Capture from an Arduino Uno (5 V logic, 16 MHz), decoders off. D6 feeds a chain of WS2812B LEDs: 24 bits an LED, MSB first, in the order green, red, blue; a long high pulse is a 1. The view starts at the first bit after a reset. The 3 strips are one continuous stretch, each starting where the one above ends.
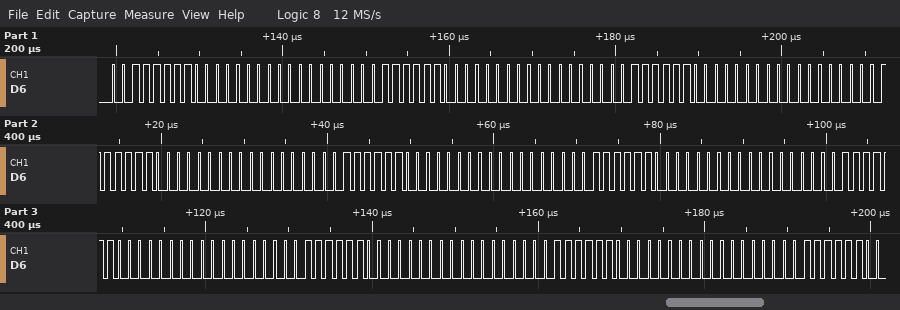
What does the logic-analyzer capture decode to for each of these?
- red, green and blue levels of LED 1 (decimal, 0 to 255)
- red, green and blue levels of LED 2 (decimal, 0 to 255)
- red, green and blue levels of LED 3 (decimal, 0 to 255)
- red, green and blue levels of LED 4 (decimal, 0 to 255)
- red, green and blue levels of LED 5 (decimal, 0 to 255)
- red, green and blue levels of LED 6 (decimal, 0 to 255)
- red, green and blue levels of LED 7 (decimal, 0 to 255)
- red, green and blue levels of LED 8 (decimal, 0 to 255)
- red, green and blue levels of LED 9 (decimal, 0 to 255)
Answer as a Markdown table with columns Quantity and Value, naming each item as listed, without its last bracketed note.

| Quantity | Value |
|---|---|
| red, green and blue levels of LED 1 | 0, 63, 0 |
| red, green and blue levels of LED 2 | 0, 63, 0 |
| red, green and blue levels of LED 3 | 0, 63, 0 |
| red, green and blue levels of LED 4 | 0, 63, 0 |
| red, green and blue levels of LED 5 | 0, 63, 0 |
| red, green and blue levels of LED 6 | 0, 63, 0 |
| red, green and blue levels of LED 7 | 0, 63, 0 |
| red, green and blue levels of LED 8 | 0, 63, 0 |
| red, green and blue levels of LED 9 | 0, 63, 0 |
